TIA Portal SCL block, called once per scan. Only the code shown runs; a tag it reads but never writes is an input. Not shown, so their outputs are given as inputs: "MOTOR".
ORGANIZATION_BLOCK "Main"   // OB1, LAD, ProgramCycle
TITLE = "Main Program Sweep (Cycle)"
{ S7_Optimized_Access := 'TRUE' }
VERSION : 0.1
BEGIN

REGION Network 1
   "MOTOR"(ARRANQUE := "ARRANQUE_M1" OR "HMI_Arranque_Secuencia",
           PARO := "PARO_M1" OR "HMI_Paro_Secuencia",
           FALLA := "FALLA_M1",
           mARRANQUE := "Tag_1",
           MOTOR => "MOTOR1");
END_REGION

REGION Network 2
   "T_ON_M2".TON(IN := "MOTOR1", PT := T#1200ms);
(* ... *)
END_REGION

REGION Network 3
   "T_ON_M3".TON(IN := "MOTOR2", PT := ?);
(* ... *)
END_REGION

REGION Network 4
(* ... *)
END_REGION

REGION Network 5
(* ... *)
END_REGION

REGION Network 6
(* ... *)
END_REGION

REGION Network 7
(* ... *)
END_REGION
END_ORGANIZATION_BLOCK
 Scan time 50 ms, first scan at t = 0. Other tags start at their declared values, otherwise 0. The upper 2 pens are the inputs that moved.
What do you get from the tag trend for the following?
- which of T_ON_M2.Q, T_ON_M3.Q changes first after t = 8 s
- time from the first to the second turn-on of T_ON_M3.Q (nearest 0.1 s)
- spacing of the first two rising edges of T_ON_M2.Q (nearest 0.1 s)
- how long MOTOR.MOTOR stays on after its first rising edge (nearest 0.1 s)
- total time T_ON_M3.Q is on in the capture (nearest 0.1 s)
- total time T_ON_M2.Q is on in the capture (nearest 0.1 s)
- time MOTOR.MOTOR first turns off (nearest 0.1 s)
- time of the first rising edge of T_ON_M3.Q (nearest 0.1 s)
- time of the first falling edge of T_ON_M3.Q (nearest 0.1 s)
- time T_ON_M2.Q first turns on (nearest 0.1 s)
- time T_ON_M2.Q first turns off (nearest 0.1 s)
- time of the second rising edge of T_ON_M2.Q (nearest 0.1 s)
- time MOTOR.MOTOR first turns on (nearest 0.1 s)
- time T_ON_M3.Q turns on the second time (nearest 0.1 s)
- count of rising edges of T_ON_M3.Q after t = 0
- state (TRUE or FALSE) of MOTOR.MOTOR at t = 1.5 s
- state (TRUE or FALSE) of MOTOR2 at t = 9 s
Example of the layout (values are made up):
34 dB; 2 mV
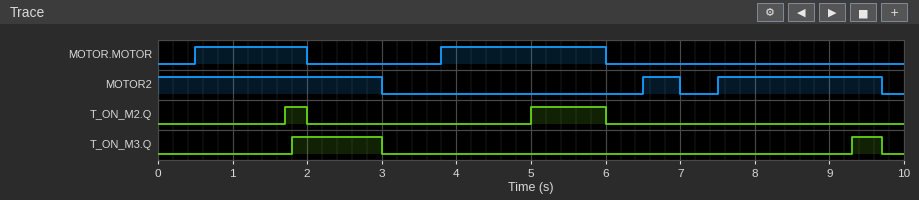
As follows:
T_ON_M3.Q; 7.5 s; 3.3 s; 1.5 s; 1.6 s; 1.3 s; 2.0 s; 1.8 s; 3.0 s; 1.7 s; 2.0 s; 5.0 s; 0.5 s; 9.3 s; 2; TRUE; TRUE
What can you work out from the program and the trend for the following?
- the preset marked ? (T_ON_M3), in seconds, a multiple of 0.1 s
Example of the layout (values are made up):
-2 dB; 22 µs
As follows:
1.8 s
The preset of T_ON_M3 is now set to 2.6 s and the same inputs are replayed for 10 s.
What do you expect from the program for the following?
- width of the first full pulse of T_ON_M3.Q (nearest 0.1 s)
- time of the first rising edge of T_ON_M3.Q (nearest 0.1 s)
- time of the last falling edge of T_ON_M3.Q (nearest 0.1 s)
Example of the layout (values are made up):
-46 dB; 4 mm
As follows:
0.4 s; 2.6 s; 3.0 s
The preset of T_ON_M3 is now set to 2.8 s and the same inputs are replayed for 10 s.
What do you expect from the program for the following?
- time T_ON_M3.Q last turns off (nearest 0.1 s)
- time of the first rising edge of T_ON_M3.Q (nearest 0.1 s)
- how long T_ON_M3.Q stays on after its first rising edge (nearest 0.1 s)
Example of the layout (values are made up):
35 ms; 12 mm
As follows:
3.0 s; 2.8 s; 0.2 s
